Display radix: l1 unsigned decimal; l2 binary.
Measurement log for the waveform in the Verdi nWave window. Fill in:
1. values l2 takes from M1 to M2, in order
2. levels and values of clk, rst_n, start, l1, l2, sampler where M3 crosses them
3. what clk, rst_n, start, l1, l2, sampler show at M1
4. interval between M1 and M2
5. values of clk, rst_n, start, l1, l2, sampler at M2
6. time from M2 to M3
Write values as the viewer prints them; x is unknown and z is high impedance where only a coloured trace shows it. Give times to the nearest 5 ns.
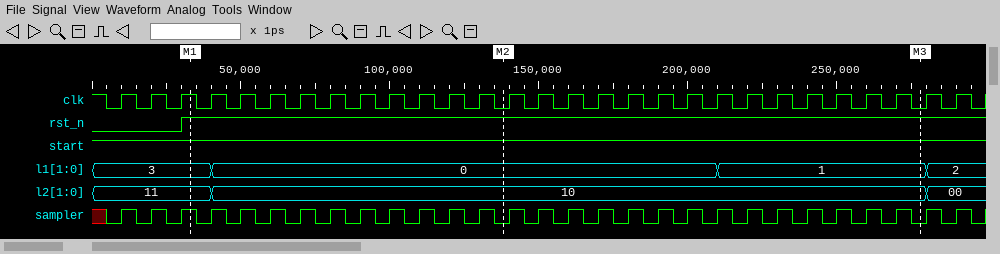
11, 10
clk=0, rst_n=1, start=1, l1=1, l2=10, sampler=0
clk=1, rst_n=1, start=1, l1=3, l2=11, sampler=1
105 ns
clk=0, rst_n=1, start=1, l1=0, l2=10, sampler=0
140 ns
